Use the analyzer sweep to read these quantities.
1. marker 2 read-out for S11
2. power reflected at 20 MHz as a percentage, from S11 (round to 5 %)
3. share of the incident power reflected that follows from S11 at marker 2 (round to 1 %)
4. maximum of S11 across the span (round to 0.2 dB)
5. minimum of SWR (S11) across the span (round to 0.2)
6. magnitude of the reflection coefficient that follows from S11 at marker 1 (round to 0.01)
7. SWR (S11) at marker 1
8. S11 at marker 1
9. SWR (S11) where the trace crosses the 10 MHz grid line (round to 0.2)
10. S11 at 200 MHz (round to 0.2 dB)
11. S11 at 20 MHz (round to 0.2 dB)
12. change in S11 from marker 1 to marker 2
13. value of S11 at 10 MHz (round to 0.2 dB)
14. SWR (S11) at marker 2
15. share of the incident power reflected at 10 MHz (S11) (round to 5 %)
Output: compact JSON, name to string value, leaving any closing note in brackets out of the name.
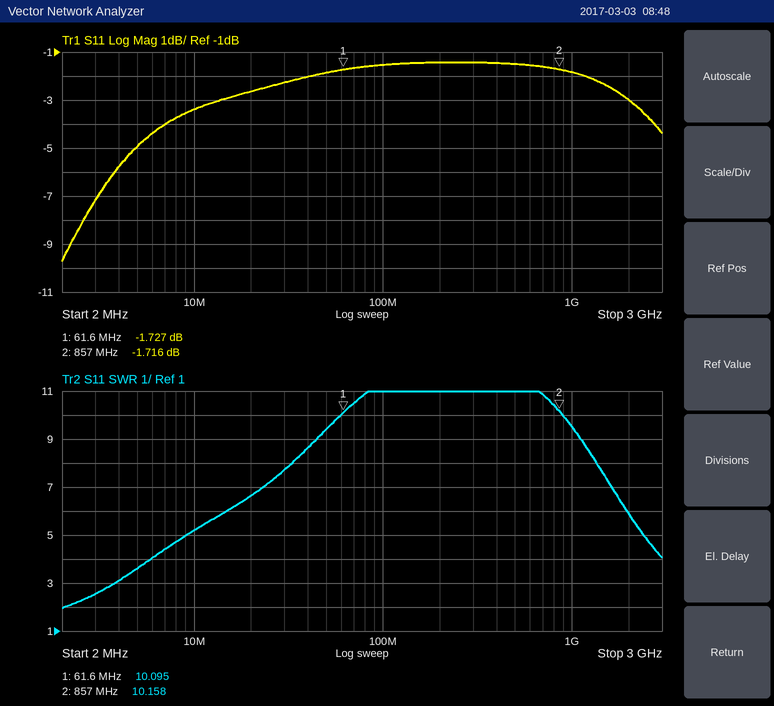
{"marker 2 read-out for S11": "-1.716 dB", "power reflected at 20 MHz as a percentage, from S11": "55 %", "share of the incident power reflected that follows from S11 at marker 2": "67 %", "maximum of S11 across the span": "-1.4 dB", "minimum of SWR (S11) across the span": "2.0", "magnitude of the reflection coefficient that follows from S11 at marker 1": "0.82", "SWR (S11) at marker 1": "10.095", "S11 at marker 1": "-1.727 dB", "SWR (S11) where the trace crosses the 10 MHz grid line": "5.2", "S11 at 200 MHz": "-1.4 dB", "S11 at 20 MHz": "-2.6 dB", "change in S11 from marker 1 to marker 2": "0.011 dB", "value of S11 at 10 MHz": "-3.4 dB", "SWR (S11) at marker 2": "10.158", "share of the incident power reflected at 10 MHz (S11)": "45 %"}
